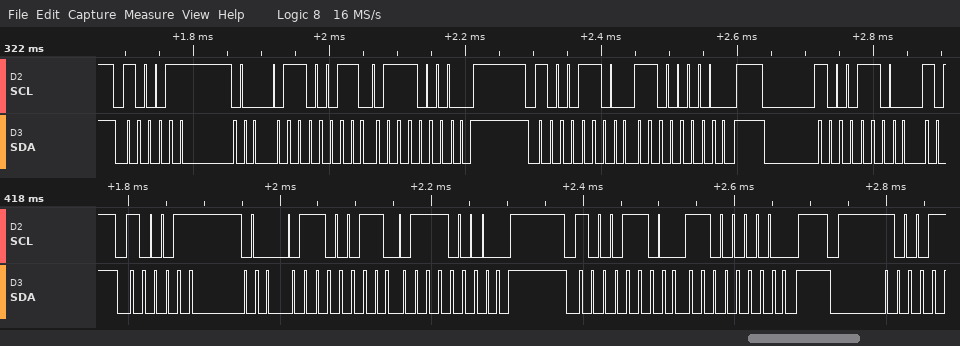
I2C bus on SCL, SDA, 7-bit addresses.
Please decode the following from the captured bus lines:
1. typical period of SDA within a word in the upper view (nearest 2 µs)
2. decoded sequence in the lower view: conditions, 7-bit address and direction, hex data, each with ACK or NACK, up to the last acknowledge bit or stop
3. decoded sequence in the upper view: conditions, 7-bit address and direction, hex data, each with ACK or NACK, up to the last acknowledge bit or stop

16 µs
start, address 46 write ACK, 63 ACK, 70 ACK, stop, start, address 46 write ACK, C0 ACK, stop
start, address 46 write ACK, 63 ACK, 70 ACK, stop, start, address 46 write ACK, C0 ACK, stop, start, address 46 write ACK
